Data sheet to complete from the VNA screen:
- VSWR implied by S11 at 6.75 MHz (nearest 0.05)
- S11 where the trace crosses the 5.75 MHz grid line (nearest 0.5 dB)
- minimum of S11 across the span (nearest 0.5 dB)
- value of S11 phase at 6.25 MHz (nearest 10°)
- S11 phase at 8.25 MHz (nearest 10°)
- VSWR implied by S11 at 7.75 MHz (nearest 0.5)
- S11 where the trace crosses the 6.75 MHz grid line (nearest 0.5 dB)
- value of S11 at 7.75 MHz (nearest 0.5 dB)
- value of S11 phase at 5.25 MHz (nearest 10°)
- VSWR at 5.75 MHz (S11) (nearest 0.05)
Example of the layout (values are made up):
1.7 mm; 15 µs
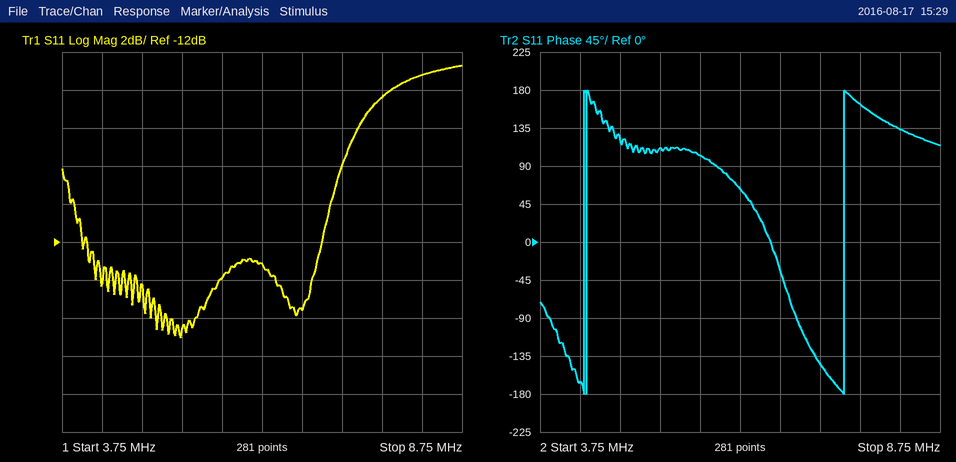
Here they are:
1.40; -14.0 dB; -17.0 dB; 60°; 130°; 4.0; -15.5 dB; -4.5 dB; 110°; 1.50
